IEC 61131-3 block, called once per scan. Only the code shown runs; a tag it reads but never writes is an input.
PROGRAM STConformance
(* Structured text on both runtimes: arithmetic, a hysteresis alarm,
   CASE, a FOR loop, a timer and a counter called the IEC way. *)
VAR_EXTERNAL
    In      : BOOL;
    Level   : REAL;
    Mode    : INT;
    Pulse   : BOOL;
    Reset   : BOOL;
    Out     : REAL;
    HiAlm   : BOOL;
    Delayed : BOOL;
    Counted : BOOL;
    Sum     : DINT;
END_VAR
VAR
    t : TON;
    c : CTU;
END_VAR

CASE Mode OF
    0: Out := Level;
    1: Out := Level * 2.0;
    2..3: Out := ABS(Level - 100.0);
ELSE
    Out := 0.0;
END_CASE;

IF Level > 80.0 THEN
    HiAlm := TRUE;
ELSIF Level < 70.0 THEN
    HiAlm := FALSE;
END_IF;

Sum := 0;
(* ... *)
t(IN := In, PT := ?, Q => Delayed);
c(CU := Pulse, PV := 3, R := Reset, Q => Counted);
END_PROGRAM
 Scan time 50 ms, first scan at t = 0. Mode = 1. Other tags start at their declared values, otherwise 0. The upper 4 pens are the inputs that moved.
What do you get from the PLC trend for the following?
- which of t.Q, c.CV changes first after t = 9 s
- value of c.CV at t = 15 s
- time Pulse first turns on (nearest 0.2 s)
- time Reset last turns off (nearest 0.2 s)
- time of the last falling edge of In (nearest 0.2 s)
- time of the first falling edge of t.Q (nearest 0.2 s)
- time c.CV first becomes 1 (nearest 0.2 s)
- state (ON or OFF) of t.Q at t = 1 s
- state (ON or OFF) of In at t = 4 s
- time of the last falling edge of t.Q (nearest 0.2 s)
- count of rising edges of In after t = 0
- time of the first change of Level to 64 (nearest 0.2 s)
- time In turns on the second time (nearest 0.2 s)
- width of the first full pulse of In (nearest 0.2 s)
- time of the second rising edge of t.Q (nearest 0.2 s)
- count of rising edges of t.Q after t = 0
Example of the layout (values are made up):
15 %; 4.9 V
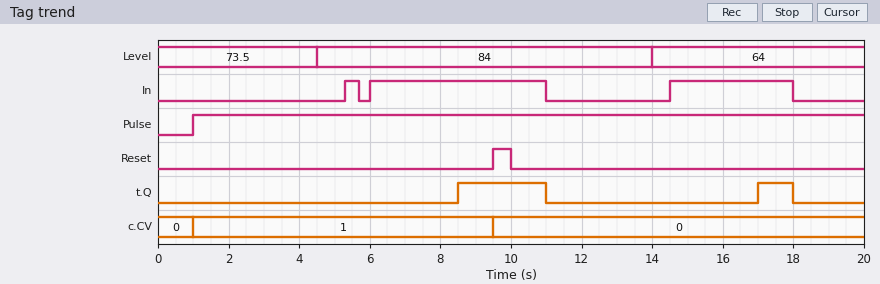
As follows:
c.CV; 0; 1.0 s; 10.0 s; 18.0 s; 11.0 s; 1.0 s; OFF; OFF; 18.0 s; 3; 14.0 s; 6.0 s; 0.4 s; 17.0 s; 2
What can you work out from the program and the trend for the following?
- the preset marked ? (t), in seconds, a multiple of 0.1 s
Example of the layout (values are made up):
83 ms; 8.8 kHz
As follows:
2.5 s
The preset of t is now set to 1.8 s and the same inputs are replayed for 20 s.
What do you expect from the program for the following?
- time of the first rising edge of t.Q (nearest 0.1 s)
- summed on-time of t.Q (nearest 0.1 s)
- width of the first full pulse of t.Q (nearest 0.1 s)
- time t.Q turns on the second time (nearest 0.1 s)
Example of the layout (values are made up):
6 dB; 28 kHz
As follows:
7.8 s; 4.9 s; 3.2 s; 16.3 s
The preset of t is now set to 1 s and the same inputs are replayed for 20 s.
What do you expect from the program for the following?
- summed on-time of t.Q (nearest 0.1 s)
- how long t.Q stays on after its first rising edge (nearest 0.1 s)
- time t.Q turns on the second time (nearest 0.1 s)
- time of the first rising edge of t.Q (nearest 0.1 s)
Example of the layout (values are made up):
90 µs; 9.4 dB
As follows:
6.5 s; 4.0 s; 15.5 s; 7.0 s
